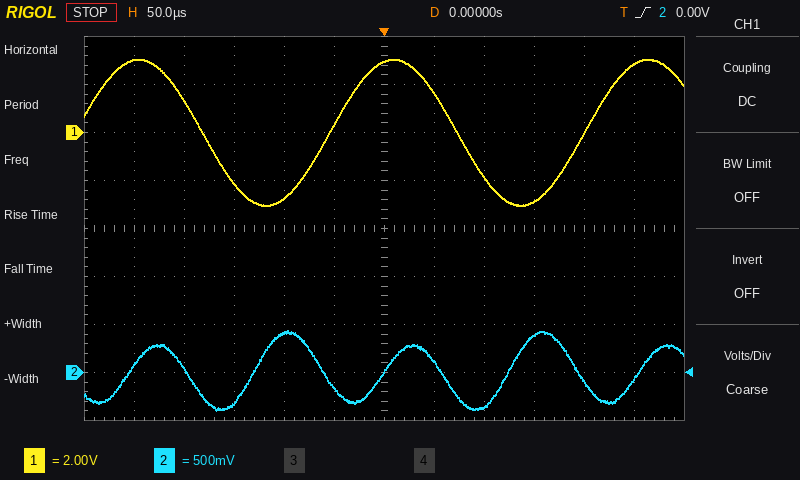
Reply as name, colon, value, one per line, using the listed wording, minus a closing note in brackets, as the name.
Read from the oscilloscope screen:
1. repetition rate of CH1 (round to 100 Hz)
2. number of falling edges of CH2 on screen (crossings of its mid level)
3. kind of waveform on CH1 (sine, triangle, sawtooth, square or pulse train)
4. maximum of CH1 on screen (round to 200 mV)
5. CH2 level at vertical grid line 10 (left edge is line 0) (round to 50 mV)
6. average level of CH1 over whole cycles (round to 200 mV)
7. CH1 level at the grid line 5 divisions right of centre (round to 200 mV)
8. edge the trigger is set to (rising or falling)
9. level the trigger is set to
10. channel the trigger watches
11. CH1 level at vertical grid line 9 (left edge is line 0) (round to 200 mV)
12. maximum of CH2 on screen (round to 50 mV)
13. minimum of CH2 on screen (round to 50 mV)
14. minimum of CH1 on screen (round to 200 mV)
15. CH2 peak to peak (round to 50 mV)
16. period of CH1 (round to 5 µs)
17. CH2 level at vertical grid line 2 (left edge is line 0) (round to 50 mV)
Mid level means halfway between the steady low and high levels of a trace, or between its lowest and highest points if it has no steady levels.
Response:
repetition rate of CH1: 3.9 kHz
number of falling edges of CH2 on screen: 4
kind of waveform on CH1: sine
maximum of CH1 on screen: 3.0 V
CH2 level at vertical grid line 10 (left edge is line 0): -100 mV
average level of CH1 over whole cycles: 0.0 V
CH1 level at the grid line 5 divisions right of centre: 2.8 V
edge the trigger is set to: rising
level the trigger is set to: 0.00 V
channel the trigger watches: CH2
CH1 level at vertical grid line 9 (left edge is line 0): -2.8 V
maximum of CH2 on screen: 450 mV
minimum of CH2 on screen: -400 mV
minimum of CH1 on screen: -3.0 V
CH2 peak to peak: 850 mV
period of CH1: 255 µs
CH2 level at vertical grid line 2 (left edge is line 0): 50 mV
